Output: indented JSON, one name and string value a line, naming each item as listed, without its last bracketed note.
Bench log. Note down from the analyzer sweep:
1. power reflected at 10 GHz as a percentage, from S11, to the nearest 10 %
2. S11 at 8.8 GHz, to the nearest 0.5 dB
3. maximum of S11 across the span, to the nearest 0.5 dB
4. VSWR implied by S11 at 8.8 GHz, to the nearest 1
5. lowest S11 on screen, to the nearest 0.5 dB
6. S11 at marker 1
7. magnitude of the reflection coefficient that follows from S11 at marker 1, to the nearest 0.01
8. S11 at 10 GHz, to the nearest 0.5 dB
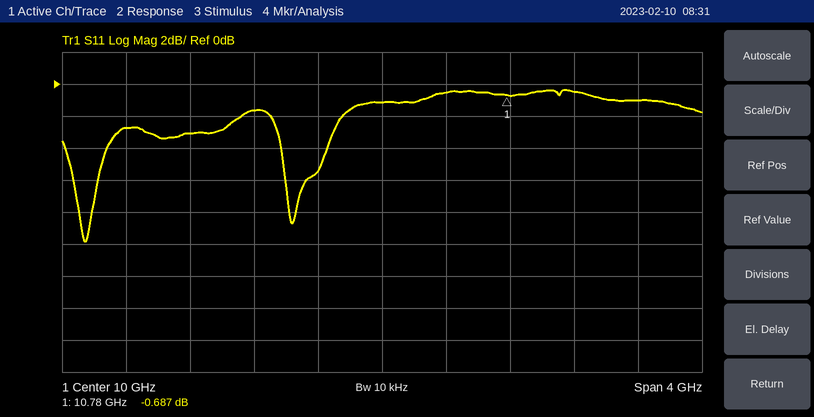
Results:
{
  "power reflected at 10 GHz as a percentage, from S11, to the nearest 10 %": "80 %",
  "S11 at 8.8 GHz, to the nearest 0.5 dB": "-3.0 dB",
  "maximum of S11 across the span, to the nearest 0.5 dB": "-0.5 dB",
  "VSWR implied by S11 at 8.8 GHz, to the nearest 1": "6",
  "lowest S11 on screen, to the nearest 0.5 dB": "-10.0 dB",
  "S11 at marker 1": "-0.687 dB",
  "magnitude of the reflection coefficient that follows from S11 at marker 1, to the nearest 0.01": "0.92",
  "S11 at 10 GHz, to the nearest 0.5 dB": "-1.0 dB"
}
